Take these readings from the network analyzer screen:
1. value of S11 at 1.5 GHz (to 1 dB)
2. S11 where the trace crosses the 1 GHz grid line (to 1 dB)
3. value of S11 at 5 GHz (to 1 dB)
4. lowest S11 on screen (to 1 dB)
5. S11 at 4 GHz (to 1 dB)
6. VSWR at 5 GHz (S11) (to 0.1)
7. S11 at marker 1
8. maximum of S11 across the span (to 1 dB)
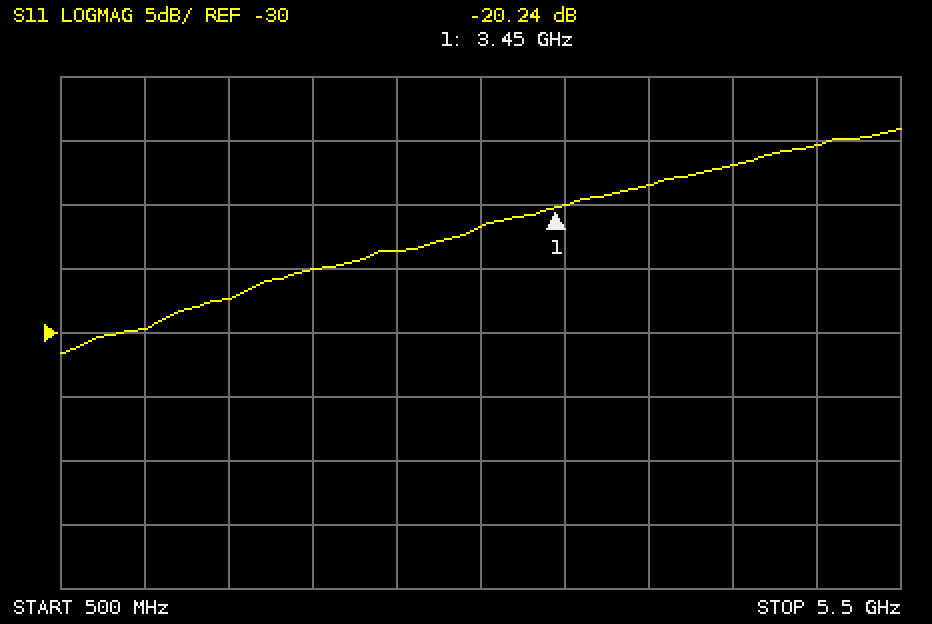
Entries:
-27 dB
-30 dB
-15 dB
-32 dB
-18 dB
1.4
-20.24 dB
-14 dB
